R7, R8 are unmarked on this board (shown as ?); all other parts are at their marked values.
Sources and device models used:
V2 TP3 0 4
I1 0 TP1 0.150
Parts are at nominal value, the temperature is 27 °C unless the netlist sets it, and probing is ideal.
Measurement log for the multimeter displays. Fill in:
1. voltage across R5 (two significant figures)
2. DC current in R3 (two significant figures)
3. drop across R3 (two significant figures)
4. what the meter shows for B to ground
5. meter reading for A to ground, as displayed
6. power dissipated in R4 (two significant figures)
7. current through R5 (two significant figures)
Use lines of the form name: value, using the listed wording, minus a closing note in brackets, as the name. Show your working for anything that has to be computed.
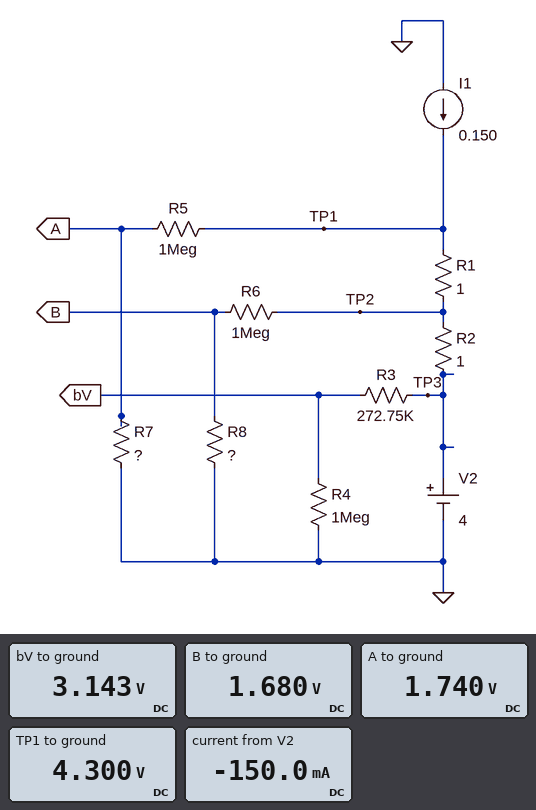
voltage across R5: 4.3 V - 1.74 V = 2.6 V
DC current in R3: (4 V - 3.143 V) / 272.8 kΩ = 3.1 µA
drop across R3: 4 V - 3.143 V = 860 mV
what the meter shows for B to ground: 1.680 V
meter reading for A to ground, as displayed: 1.740 V
power dissipated in R4: (3.143 V)^2 / 1 MΩ = 9.9 µW
current through R5: (4.3 V - 1.74 V) / 1 MΩ = 2.6 µA
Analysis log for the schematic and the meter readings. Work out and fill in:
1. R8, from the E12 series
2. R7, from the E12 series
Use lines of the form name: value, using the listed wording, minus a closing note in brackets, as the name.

R8, from the E12 series: 680 kΩ
R7, from the E12 series: 680 kΩ
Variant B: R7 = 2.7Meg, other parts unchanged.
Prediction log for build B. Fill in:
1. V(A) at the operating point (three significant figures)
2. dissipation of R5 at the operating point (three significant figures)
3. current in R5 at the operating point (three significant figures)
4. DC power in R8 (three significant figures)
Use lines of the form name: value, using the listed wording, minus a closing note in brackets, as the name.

V(A) at the operating point: 3.14 V
dissipation of R5 at the operating point: 1.35 µW
current in R5 at the operating point: 1.16 µA
DC power in R8: 4.15 µW
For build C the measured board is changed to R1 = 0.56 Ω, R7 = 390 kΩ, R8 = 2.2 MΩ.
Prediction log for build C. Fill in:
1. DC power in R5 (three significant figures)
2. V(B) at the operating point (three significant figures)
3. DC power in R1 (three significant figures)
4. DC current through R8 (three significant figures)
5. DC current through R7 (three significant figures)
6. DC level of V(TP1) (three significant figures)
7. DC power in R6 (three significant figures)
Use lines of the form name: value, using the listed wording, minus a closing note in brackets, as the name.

DC power in R5: 9.28 µW
V(B) at the operating point: 2.85 V
DC power in R1: 12.6 mW
DC current through R8: 1.30 µA
DC current through R7: 3.05 µA
DC level of V(TP1): 4.23 V
DC power in R6: 1.68 µW
